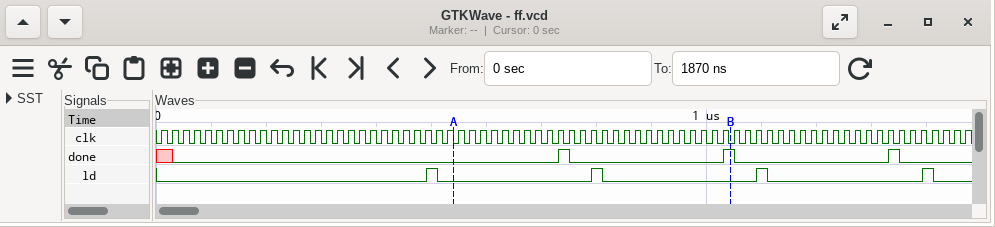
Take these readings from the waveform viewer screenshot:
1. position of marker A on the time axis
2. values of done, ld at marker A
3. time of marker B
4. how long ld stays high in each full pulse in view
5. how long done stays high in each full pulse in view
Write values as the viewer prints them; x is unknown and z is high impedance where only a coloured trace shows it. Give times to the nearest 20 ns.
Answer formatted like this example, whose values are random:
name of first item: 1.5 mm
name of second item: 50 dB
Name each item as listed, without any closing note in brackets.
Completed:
position of marker A on the time axis: 540 ns
values of done, ld at marker A: done=0, ld=0
time of marker B: 1040 ns
how long ld stays high in each full pulse in view: 20 ns, 20 ns, 20 ns, 20 ns
how long done stays high in each full pulse in view: 20 ns, 20 ns, 20 ns
